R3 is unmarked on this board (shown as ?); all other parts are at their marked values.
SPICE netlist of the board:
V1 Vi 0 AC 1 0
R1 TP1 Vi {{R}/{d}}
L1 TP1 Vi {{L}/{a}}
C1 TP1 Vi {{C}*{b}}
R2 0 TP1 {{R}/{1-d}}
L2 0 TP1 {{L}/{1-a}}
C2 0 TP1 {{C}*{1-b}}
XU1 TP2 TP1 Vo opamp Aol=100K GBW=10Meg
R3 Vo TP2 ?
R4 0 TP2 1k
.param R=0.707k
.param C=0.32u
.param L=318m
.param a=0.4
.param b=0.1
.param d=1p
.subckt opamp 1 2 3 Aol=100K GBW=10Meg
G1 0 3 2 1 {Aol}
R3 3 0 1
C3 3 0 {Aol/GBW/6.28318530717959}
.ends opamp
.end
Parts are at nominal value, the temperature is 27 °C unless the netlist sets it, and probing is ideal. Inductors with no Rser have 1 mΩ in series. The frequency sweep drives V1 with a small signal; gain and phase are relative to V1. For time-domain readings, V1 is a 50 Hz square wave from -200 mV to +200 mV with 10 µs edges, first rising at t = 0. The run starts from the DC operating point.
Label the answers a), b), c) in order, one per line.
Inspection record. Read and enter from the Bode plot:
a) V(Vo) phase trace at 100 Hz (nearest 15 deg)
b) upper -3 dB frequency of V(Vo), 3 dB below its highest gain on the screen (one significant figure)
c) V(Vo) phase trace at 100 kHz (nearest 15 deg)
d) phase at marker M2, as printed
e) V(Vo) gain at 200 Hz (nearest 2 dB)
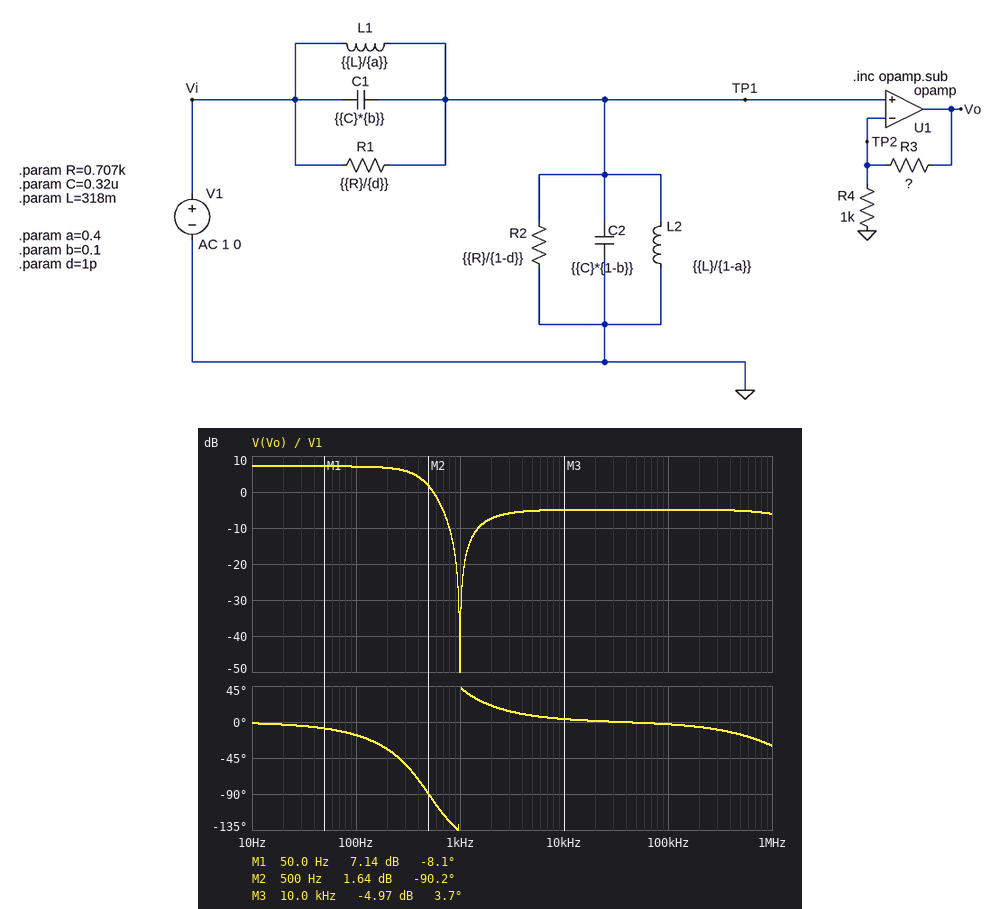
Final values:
a) -15 deg
b) 400 Hz
c) 0 deg
d) -90.2 deg
e) 6 dB
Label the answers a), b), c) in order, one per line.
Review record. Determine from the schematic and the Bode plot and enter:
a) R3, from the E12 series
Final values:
a) 4.7 kΩ
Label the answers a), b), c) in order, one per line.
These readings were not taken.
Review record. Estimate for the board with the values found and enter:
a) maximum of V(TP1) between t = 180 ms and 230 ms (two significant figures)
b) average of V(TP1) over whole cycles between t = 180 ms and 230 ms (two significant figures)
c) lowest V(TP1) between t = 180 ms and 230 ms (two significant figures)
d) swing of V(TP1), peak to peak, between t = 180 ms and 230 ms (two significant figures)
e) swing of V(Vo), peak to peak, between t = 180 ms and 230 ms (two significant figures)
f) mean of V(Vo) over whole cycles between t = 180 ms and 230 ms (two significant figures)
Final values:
a) 66 mV
b) -20 mV
c) -110 mV
d) 170 mV
e) 980 mV
f) -110 mV
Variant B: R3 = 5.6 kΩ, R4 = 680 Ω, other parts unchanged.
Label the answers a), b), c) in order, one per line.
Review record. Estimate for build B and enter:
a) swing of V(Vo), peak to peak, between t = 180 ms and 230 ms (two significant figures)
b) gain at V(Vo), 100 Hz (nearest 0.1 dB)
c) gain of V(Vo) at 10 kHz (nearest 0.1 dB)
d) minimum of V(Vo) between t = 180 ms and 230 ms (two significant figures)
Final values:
a) 1.6 V
b) 11.3 dB
c) -0.8 dB
d) -980 mV
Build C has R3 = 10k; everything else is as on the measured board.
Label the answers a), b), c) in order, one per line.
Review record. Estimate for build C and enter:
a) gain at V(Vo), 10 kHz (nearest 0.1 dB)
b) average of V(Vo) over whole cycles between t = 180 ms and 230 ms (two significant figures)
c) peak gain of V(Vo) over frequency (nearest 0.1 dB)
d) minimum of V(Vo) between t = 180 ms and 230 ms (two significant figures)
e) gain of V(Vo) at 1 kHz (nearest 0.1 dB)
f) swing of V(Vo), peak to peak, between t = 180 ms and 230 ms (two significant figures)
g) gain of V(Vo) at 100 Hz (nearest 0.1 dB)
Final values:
a) 0.7 dB
b) -220 mV
c) 12.9 dB
d) -1.2 V
e) -46.7 dB
f) 1.9 V
g) 12.8 dB
